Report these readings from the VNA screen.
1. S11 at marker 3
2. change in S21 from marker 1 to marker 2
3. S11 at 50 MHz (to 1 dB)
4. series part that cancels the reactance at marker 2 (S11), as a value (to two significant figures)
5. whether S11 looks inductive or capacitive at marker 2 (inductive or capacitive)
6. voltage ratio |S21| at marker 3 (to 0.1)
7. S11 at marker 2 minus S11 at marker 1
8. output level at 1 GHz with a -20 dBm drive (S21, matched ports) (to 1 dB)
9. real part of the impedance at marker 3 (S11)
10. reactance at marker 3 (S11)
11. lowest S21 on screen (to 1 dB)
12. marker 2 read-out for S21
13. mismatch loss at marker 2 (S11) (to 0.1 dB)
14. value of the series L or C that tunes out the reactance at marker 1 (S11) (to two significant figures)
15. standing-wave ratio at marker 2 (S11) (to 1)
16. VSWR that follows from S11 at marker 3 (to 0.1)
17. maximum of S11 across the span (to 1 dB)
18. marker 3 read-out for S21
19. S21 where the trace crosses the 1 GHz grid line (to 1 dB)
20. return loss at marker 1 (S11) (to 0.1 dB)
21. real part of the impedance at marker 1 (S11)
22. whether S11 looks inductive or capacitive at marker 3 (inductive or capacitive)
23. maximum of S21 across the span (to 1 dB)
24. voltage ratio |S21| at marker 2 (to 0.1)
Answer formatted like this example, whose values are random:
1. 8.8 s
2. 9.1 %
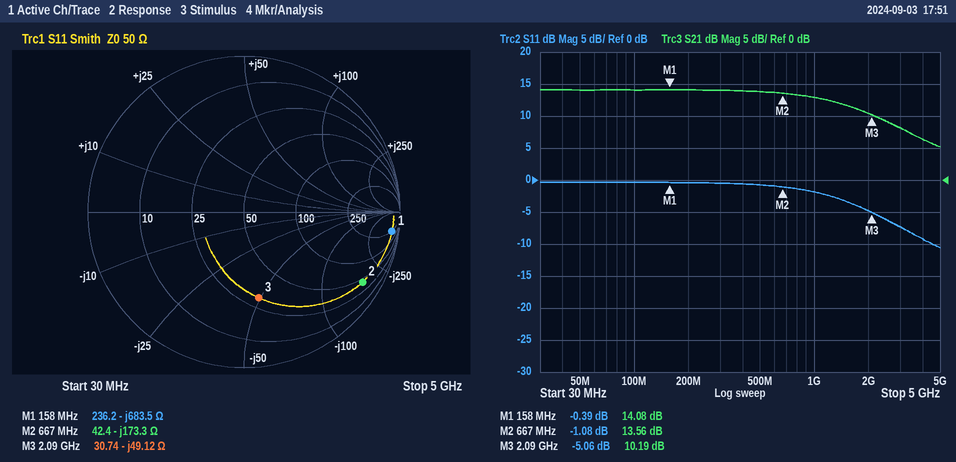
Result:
1. -5.06 dB
2. -0.52 dB
3. 0 dB
4. 41 nH
5. capacitive
6. 3.2
7. -0.69 dB
8. -7 dBm
9. 30.74 Ω
10. -49.12 Ω
11. 5 dB
12. 13.56 dB
13. 6.6 dB
14. 690 nH
15. 16
16. 3.5
17. 0 dB
18. 10.19 dB
19. 13 dB
20. 0.4 dB
21. 236.2 Ω
22. capacitive
23. 14 dB
24. 4.8
